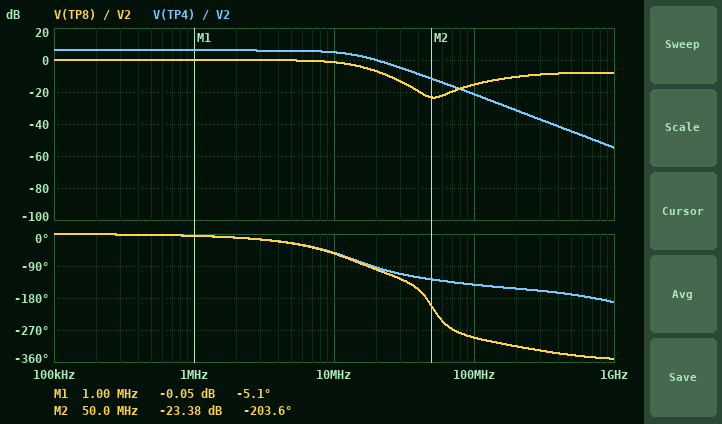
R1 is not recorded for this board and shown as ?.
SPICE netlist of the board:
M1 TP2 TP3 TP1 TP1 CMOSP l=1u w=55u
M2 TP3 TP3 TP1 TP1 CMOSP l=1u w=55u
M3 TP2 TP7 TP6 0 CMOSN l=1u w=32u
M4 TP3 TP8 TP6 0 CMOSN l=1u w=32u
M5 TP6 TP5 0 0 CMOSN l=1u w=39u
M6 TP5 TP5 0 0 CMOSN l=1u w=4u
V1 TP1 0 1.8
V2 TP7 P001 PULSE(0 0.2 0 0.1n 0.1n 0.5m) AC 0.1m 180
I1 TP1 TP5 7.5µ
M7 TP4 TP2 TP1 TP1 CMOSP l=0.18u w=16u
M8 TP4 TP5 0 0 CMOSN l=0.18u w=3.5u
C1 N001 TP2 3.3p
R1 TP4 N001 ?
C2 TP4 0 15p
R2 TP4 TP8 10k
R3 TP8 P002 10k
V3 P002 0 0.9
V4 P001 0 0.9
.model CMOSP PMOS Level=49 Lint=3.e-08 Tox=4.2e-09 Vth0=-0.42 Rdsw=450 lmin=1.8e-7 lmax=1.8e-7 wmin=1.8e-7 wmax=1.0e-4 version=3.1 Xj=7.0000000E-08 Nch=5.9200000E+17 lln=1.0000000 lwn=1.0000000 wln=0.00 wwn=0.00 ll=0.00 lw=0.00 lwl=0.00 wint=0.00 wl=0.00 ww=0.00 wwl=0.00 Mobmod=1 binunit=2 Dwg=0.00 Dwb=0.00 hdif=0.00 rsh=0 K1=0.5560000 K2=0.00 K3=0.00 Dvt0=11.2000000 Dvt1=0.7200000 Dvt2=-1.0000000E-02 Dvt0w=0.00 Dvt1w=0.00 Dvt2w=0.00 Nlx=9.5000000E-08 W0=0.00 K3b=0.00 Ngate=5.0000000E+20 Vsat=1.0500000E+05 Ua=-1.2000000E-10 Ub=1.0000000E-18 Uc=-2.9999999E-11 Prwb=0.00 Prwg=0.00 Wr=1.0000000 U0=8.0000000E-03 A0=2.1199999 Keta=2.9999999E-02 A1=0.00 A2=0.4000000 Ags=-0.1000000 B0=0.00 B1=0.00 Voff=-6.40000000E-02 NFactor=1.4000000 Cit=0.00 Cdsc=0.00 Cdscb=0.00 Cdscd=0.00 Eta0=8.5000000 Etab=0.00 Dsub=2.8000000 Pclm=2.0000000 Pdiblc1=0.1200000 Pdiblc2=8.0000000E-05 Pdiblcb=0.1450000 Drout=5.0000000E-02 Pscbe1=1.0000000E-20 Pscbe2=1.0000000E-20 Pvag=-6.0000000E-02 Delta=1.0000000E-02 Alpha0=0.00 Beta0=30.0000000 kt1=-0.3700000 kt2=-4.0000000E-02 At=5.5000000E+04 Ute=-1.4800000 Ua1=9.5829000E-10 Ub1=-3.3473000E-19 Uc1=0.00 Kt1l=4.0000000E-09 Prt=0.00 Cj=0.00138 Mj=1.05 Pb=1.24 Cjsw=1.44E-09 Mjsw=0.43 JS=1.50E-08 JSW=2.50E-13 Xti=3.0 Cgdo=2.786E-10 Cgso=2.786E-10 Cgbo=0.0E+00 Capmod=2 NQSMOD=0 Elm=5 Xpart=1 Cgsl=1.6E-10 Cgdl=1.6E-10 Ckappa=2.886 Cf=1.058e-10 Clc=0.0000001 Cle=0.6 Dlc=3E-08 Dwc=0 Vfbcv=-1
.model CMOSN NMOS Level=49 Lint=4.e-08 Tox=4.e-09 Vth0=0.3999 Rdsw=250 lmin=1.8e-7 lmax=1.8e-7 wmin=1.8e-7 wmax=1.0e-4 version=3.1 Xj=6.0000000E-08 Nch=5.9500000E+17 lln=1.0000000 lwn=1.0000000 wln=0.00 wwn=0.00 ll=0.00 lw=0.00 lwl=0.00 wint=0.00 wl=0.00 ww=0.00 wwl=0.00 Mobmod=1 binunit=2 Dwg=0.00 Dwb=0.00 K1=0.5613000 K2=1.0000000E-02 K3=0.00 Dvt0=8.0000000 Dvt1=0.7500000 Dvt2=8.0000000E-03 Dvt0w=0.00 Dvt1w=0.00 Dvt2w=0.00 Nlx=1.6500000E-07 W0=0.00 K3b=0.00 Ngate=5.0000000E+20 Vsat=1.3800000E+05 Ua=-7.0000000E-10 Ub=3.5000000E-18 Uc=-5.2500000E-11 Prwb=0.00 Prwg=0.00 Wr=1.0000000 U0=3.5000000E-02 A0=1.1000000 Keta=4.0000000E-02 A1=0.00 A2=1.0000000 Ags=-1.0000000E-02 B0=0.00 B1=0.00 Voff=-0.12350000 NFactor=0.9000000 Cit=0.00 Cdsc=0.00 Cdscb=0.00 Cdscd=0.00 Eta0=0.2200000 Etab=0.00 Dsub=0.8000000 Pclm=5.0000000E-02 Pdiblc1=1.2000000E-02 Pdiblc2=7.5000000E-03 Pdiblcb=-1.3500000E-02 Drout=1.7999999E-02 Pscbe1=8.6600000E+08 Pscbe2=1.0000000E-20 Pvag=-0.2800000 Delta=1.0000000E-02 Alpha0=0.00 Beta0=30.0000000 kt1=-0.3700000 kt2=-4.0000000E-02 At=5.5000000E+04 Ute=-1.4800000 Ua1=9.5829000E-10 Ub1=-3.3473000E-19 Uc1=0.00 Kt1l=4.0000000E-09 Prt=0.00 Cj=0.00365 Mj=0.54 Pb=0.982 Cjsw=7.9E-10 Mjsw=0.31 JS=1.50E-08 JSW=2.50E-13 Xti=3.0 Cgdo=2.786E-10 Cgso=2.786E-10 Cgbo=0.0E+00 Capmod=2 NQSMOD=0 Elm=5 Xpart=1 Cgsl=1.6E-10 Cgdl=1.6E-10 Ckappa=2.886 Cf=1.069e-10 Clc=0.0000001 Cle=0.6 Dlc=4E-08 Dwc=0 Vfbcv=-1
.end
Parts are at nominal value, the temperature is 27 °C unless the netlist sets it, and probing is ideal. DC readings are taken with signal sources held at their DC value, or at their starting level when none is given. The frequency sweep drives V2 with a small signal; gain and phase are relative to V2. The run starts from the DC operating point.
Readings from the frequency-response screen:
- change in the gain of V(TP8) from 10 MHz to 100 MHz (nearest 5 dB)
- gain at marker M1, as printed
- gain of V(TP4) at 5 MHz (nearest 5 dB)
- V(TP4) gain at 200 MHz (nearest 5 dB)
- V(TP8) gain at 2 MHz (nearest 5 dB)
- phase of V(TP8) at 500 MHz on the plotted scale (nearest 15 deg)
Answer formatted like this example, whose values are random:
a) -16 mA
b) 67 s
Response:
a) -15 dB
b) -0.05 dB
c) 5 dB
d) -30 dB
e) 0 dB
f) -345 deg
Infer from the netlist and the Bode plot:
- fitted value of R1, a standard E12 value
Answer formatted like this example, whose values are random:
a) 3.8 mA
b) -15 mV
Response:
a) 2.2 kΩ
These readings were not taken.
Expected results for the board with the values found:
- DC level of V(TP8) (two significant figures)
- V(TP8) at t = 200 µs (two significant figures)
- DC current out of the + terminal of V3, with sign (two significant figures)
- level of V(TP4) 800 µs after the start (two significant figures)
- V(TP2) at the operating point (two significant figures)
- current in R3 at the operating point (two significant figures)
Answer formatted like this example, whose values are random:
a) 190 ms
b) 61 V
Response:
a) 900 mV
b) 1.1 V
c) -310 nA
d) 910 mV
e) 1.4 V
f) 310 nA
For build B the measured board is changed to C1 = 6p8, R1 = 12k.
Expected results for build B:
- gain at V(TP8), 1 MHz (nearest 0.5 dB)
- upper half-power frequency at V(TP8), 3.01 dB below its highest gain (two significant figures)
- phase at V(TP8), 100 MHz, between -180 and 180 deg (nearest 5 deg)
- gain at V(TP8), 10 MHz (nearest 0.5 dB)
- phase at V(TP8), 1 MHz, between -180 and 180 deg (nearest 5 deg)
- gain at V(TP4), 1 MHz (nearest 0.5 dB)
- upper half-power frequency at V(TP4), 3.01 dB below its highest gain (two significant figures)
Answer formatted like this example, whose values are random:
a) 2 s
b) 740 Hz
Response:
a) -0.5 dB
b) 57 MHz
c) 110 deg
d) -2.5 dB
e) -10 deg
f) 5.5 dB
g) 60 MHz
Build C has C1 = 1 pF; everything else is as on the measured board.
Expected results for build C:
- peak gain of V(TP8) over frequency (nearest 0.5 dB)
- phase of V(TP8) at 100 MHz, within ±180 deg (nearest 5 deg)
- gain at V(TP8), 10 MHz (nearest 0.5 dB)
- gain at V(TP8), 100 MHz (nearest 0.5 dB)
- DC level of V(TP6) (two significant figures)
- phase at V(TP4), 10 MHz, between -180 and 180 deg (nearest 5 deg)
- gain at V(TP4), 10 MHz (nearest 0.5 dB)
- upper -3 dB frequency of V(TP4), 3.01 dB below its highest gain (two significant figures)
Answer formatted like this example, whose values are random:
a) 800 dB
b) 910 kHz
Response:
a) 4.5 dB
b) 75 deg
c) 1.0 dB
d) -14.5 dB
e) 310 mV
f) -20 deg
g) 7.5 dB
h) 28 MHz
